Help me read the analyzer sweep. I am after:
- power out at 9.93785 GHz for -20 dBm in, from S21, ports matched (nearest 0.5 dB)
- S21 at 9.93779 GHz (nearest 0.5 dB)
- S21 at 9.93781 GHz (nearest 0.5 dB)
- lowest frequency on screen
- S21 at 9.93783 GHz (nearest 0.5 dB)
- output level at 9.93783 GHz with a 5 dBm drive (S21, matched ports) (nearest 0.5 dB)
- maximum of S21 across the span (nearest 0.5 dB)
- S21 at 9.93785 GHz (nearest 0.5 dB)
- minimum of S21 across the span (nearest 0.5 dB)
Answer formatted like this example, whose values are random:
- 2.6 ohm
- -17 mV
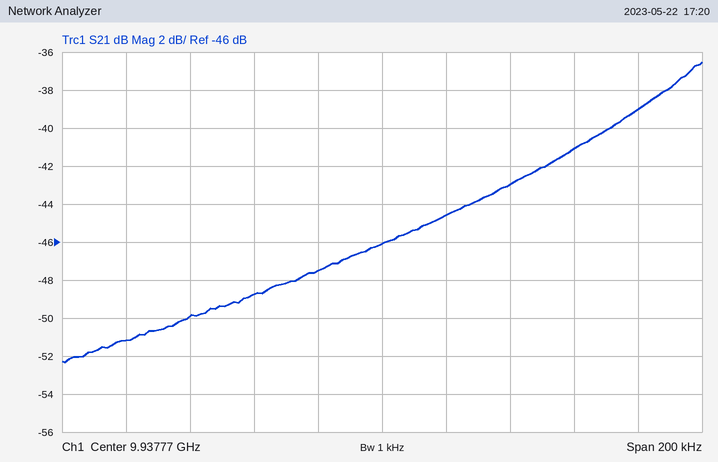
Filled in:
- -59.0 dBm
- -44.5 dB
- -43.0 dB
- 9.93767 GHz
- -41.0 dB
- -36.0 dBm
- -36.5 dB
- -39.0 dB
- -52.5 dB
